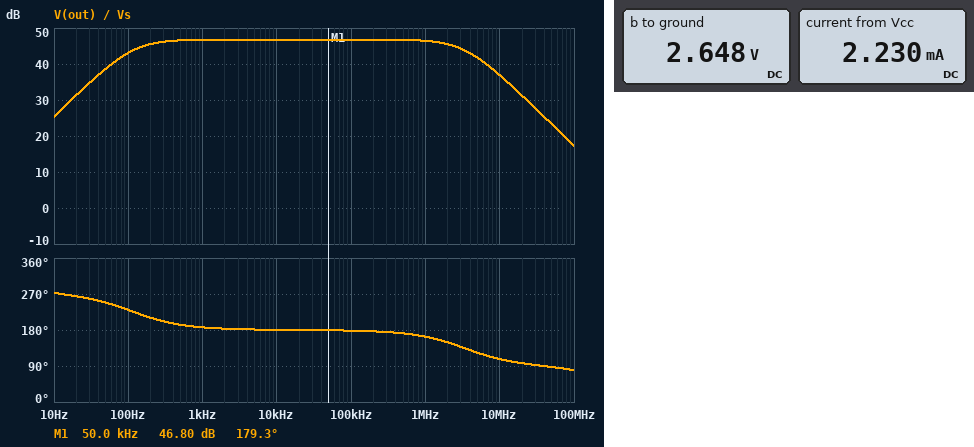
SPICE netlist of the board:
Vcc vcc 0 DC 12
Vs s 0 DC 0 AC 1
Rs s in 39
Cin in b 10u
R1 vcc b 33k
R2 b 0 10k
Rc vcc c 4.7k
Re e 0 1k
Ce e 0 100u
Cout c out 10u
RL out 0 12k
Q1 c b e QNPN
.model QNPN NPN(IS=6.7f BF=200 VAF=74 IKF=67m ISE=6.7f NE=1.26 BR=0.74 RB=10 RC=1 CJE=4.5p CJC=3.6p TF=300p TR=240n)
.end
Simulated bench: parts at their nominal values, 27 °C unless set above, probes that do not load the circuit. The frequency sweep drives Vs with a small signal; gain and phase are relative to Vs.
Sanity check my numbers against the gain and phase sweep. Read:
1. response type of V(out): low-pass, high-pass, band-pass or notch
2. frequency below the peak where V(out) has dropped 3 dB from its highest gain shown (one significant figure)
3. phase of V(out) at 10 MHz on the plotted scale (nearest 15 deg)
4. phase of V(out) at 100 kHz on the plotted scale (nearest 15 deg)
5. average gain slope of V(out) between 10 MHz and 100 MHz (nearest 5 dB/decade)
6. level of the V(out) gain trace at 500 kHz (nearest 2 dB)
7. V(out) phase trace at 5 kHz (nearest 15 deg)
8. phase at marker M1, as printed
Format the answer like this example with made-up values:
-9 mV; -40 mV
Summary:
band-pass; 100 Hz; 105 deg; 180 deg; -20 dB/decade; 46 dB; 180 deg; 179.3 deg
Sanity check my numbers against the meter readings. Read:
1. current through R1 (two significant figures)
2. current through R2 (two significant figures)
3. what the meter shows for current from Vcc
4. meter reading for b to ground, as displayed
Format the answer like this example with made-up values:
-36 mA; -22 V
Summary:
280 µA; 260 µA; 2.230 mA; 2.648 V
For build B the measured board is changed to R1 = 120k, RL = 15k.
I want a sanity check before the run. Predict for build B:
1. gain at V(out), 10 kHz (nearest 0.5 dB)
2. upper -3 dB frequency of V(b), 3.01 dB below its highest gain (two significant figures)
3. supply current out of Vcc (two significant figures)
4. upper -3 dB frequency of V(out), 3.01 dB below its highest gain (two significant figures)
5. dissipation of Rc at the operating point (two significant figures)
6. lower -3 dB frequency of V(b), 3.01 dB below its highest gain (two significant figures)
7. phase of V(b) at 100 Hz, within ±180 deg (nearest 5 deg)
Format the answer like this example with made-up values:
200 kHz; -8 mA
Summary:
31.0 dB; 120 MHz; 360 µA; 19 MHz; 330 µW; 2.0 Hz; 0 deg
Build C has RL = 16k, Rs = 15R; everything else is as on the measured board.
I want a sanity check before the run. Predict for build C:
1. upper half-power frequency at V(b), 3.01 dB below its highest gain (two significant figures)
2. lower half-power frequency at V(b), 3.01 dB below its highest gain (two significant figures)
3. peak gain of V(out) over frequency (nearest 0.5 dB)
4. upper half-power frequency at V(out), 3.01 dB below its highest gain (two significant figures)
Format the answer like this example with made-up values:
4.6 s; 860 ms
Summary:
10 MHz; 2.4 Hz; 47.5 dB; 5.1 MHz
